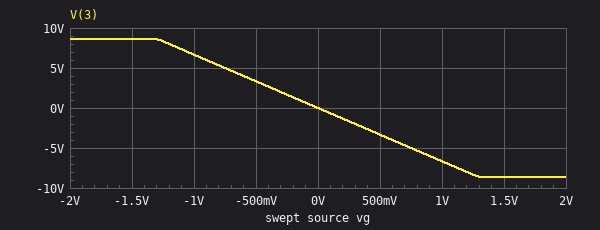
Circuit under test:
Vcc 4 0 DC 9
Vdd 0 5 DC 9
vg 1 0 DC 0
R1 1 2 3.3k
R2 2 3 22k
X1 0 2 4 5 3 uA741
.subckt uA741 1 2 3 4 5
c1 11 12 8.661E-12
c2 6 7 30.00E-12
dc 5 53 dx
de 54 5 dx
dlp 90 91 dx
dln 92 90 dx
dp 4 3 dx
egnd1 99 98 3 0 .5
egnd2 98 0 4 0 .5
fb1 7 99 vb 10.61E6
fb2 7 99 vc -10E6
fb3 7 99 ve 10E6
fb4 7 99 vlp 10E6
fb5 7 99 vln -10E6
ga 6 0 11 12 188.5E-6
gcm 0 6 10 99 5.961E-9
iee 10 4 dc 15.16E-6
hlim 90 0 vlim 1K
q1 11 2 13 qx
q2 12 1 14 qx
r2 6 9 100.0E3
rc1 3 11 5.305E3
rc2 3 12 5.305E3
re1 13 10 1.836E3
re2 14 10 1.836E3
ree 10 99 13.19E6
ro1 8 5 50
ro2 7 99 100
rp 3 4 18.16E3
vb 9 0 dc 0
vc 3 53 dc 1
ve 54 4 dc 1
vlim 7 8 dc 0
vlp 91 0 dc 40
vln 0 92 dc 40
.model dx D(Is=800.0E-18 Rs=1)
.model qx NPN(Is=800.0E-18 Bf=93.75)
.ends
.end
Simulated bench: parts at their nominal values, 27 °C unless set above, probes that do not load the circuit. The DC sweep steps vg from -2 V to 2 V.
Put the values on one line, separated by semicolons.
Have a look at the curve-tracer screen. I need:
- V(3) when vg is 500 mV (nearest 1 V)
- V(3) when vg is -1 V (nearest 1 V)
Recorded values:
-3 V; 7 V
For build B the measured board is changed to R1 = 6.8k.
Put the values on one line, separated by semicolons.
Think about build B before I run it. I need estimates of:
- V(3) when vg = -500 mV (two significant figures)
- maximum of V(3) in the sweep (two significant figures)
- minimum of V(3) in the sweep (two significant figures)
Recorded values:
1.6 V; 6.5 V; -6.5 V
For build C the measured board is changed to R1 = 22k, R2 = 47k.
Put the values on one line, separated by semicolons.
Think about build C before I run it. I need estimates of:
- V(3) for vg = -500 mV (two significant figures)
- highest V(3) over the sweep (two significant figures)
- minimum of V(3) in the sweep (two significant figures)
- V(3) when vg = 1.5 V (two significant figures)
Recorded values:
1.1 V; 4.3 V; -4.3 V; -3.2 V
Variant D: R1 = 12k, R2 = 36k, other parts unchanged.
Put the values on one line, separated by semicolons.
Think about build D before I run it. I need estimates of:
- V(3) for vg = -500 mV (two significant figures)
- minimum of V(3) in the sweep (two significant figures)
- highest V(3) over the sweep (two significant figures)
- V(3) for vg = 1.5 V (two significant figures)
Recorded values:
1.5 V; -6.0 V; 6.0 V; -4.5 V
